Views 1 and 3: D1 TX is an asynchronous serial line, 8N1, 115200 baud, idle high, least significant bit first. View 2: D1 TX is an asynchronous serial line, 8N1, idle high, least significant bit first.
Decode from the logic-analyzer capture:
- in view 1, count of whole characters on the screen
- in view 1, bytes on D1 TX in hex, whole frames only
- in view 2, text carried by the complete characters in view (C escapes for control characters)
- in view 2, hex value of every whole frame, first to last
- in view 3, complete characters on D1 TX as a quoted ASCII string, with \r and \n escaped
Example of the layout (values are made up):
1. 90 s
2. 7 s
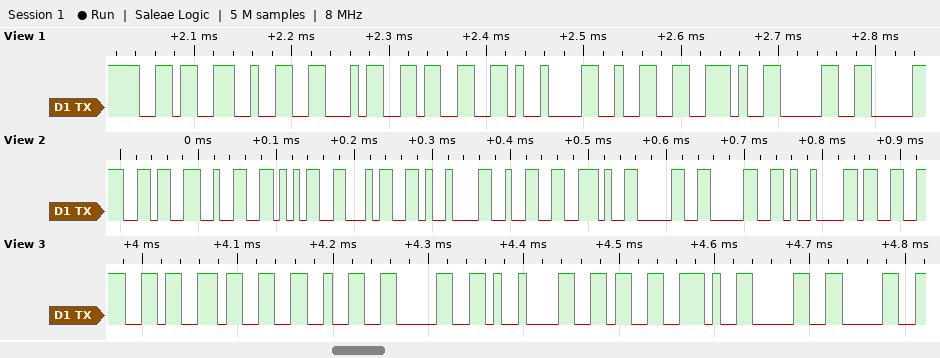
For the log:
1. 8
2. 36 32 34 33 09 32 2E 30
3. "6254\t2.00\t3"
4. 36 32 35 34 09 32 2E 30 30 09 33
5. "6320\t6.00"
